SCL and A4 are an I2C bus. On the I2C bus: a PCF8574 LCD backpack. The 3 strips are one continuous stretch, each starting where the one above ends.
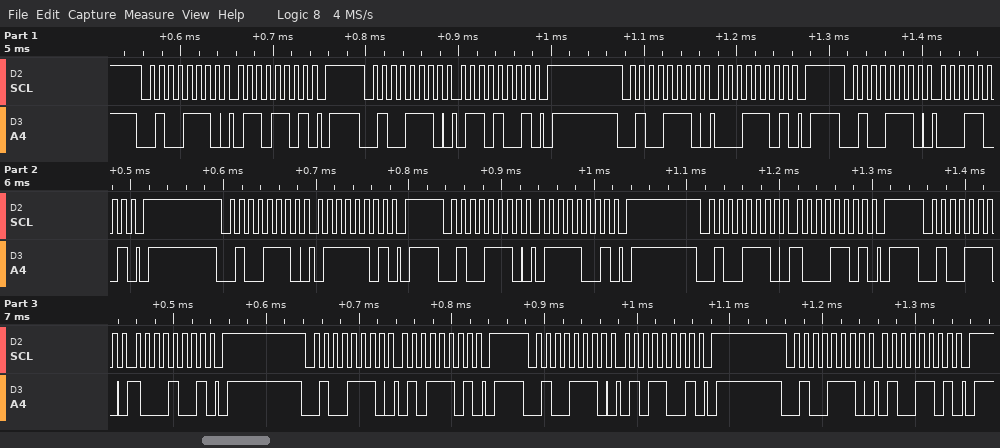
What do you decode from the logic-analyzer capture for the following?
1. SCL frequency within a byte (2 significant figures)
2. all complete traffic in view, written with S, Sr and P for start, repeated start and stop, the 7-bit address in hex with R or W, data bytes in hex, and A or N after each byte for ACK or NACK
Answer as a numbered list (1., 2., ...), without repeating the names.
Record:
1. 100 kHz
2. S 27W A 6D A P S 27W A 69 A P S 27W A 1D A P S 27W A 19 A P S 27W A 7D A P S 27W A 79 A P S 27W A 8D A P S 27W A 89 A P S 27W A 5D A P S 27W A 59 A P S 27W A 4D A P
